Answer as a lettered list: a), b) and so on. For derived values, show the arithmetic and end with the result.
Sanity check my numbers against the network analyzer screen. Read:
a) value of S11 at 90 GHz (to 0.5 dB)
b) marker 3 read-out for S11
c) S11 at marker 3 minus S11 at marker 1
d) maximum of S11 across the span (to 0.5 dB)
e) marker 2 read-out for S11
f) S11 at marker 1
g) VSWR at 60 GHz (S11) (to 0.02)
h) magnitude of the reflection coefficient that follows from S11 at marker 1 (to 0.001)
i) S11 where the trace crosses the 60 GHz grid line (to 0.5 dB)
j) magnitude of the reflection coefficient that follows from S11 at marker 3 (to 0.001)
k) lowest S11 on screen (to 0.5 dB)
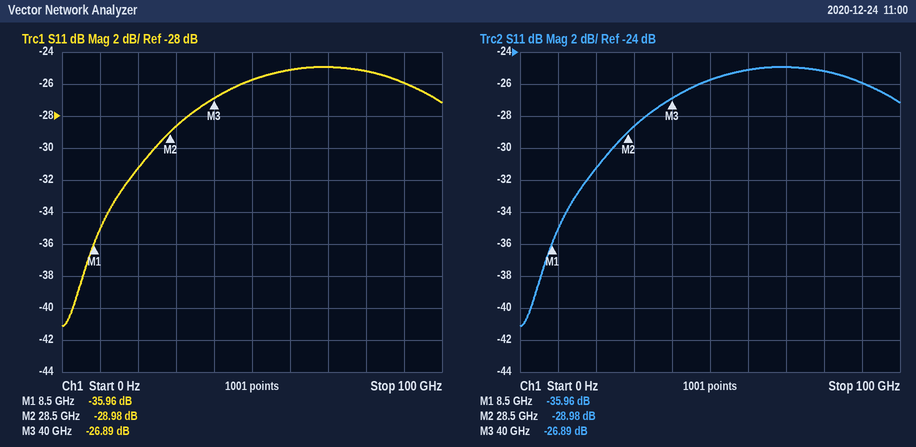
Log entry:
a) -26.0 dB
b) -26.89 dB
c) -26.89 − (-35.96) = 9.07 dB
d) -25.0 dB
e) -28.98 dB
f) -35.96 dB
g) |Γ| = 10^(-25/20) = 0.0562; VSWR = (1 + 0.0562)/(1 − 0.0562) ≈ 1.12
h) 10^(-35.96/20) ≈ 0.016
i) -25.0 dB
j) 10^(-26.89/20) ≈ 0.045
k) -41.0 dB
